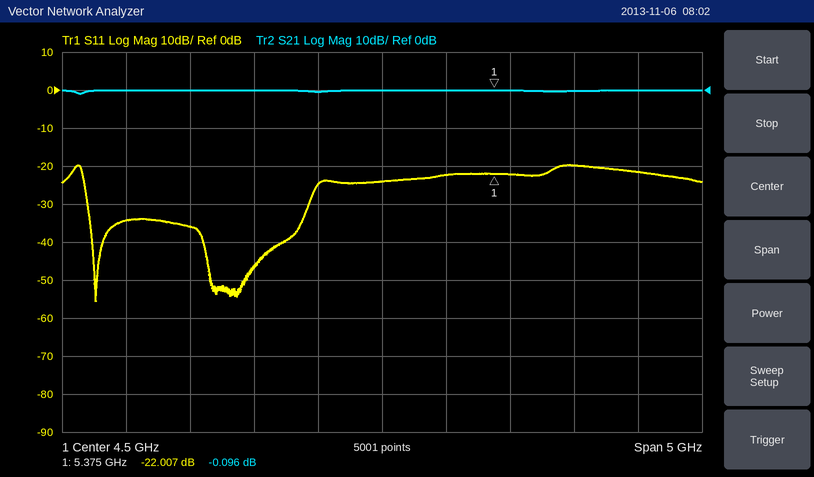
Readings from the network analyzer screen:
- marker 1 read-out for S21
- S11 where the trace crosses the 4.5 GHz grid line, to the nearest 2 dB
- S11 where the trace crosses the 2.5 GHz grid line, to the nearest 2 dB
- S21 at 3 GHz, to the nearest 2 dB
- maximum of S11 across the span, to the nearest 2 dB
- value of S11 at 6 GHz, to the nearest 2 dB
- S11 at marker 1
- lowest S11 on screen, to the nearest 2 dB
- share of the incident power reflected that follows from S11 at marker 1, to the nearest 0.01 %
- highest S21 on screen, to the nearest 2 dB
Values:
-0.096 dB
-24 dB
-34 dB
0 dB
-20 dB
-20 dB
-22.007 dB
-56 dB
0.63 %
0 dB
